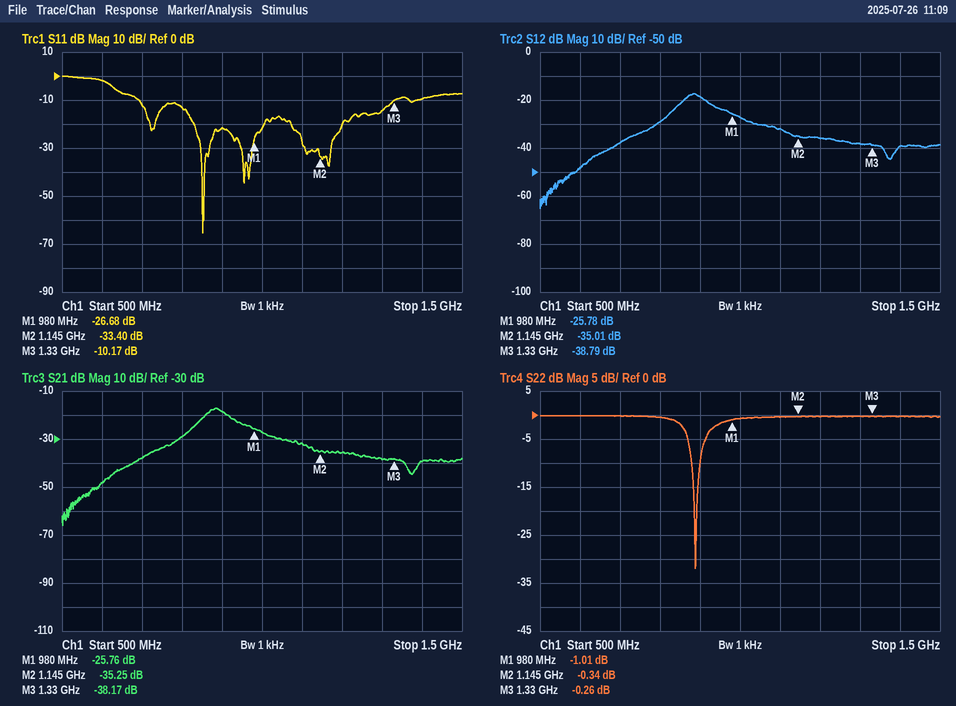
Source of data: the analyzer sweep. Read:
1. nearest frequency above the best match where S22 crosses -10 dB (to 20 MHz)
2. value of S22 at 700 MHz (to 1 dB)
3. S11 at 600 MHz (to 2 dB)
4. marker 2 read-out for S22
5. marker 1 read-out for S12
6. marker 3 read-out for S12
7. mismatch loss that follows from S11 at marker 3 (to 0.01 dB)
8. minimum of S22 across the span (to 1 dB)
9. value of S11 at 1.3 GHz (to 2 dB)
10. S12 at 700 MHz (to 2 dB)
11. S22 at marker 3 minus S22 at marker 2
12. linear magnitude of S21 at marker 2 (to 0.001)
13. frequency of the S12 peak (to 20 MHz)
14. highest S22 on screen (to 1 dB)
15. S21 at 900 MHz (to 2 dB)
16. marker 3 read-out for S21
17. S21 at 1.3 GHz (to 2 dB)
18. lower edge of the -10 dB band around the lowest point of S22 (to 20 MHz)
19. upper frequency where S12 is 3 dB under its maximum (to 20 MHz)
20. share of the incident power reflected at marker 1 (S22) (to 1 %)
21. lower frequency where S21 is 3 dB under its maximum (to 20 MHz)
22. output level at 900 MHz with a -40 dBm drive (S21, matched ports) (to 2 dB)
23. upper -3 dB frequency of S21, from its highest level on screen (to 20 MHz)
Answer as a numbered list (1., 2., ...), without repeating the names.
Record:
1. 900 MHz
2. 0 dB
3. -2 dB
4. -0.34 dB
5. -25.78 dB
6. -38.79 dB
7. 0.44 dB
8. -32 dB
9. -14 dB
10. -38 dB
11. 0.08 dB
12. 0.017
13. 880 MHz
14. 0 dB
15. -18 dB
16. -38.17 dB
17. -38 dB
18. 880 MHz
19. 920 MHz
20. 79 %
21. 860 MHz
22. -58 dBm
23. 920 MHz
